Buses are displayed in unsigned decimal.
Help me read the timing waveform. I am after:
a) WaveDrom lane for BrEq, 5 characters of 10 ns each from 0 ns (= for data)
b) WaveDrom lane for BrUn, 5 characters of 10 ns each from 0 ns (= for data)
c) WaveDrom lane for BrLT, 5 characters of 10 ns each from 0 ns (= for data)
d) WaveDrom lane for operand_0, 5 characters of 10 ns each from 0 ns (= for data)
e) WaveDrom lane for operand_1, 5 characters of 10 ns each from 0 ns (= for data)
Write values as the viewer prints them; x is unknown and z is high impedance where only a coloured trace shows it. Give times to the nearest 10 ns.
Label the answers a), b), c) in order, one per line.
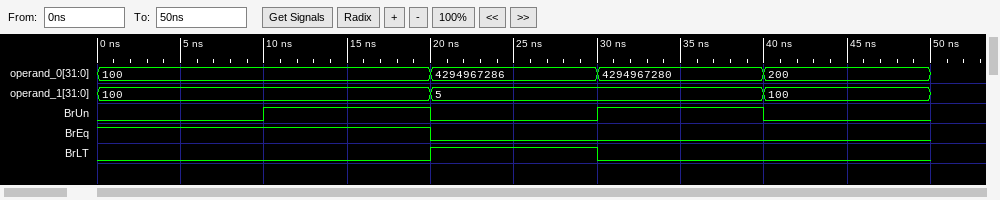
a) {name: 'BrEq', wave: '1.0..'}
b) {name: 'BrUn', wave: '01010'}
c) {name: 'BrLT', wave: '0.10.'}
d) {name: 'operand_0', wave: '=.===', data: '100 4294967286 4294967280 200'}
e) {name: 'operand_1', wave: '=.=.=', data: '100 5 100'}
